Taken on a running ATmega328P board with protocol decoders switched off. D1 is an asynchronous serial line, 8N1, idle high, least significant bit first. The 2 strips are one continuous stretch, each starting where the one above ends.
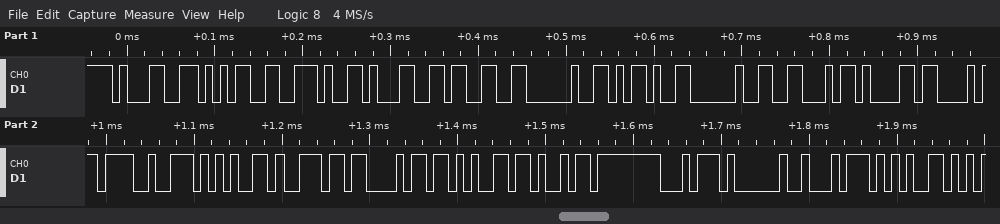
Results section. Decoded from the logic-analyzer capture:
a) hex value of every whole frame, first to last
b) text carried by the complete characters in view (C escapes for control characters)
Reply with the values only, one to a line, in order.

31 35 2E 31 33 20 2D 20 46 61 68 72 65 6E 68 65 69 74 20 74 65
"15.13 - Fahrenheit te"
